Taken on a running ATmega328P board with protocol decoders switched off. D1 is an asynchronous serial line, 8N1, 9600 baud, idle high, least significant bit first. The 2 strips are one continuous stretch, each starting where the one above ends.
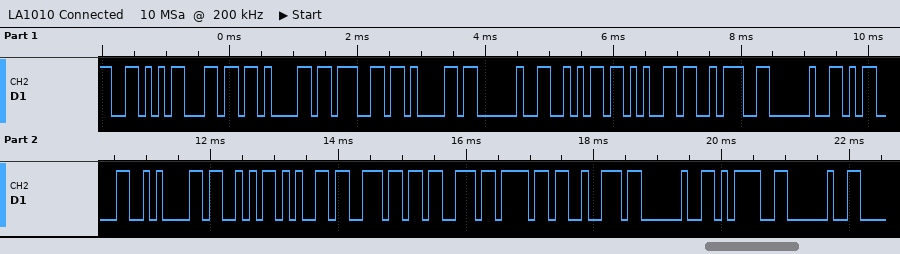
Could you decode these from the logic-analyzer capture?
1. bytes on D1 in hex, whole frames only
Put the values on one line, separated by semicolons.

56 6C 61 67 61 20 6A 65 3A 20 0D 0A 53 65 6E 73 6F 72 20 3D 20
